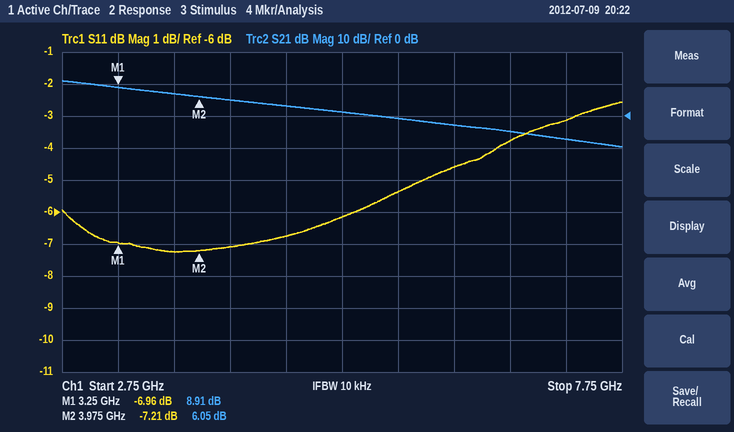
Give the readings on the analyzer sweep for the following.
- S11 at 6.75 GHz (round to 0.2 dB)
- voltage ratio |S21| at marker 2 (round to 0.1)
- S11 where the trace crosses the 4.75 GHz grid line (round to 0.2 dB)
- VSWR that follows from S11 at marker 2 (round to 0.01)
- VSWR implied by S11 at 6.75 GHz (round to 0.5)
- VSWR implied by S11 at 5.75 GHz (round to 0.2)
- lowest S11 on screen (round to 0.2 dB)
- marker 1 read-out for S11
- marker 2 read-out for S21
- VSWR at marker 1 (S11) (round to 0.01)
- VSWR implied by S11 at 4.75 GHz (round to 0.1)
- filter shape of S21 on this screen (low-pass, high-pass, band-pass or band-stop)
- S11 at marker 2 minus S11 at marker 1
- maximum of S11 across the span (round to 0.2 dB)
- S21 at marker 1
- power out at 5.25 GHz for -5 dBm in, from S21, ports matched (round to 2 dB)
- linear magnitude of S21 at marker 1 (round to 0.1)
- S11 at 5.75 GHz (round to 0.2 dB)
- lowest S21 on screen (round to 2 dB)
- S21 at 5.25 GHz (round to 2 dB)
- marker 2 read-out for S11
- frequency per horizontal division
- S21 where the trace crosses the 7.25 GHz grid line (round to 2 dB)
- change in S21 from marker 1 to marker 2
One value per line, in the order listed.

-3.8 dB
2.0
-6.8 dB
2.55
4.5
3.4
-7.2 dB
-6.96 dB
6.05 dB
2.63
2.7
low-pass
-0.25 dB
-2.6 dB
8.91 dB
-4 dBm
2.8
-5.4 dB
-10 dB
2 dB
-7.21 dB
500 MHz
-8 dB
-2.86 dB
